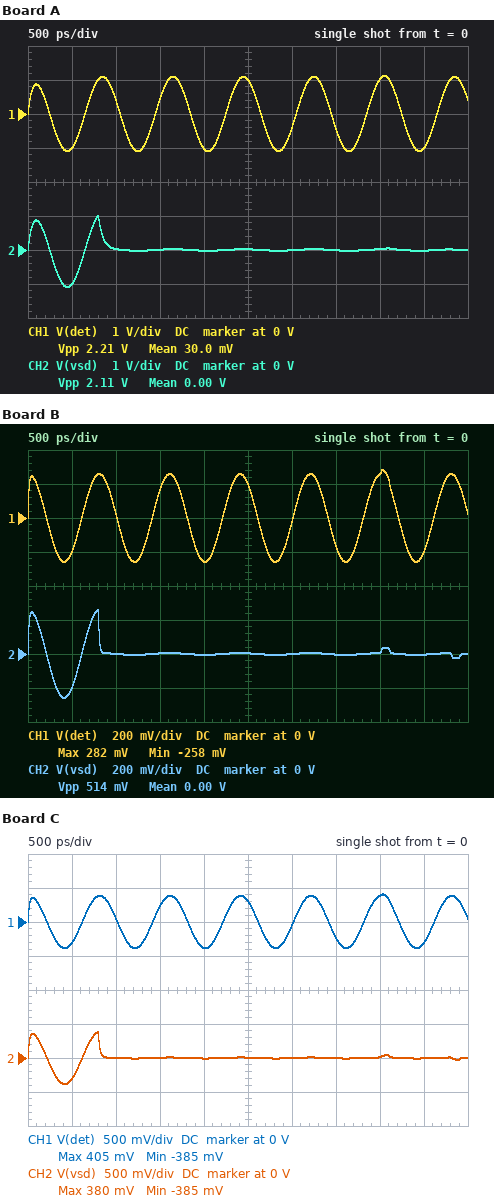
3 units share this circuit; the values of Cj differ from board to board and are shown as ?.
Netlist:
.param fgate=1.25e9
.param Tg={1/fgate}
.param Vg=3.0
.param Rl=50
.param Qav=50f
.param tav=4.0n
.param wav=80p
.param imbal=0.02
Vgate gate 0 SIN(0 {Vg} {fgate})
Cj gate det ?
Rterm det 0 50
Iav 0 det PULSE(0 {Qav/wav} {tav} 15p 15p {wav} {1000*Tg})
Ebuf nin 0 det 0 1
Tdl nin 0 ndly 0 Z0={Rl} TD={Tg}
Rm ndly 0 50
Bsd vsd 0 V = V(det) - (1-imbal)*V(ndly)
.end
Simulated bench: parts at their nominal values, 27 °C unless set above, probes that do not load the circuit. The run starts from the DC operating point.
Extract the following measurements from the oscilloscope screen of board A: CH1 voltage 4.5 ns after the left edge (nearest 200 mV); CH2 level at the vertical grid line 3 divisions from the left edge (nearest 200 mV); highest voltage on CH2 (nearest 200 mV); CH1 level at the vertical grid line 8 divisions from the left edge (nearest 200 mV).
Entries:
-1.0 V
0 V
1.0 V
1.0 V
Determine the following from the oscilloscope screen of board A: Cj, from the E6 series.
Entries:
1 pF
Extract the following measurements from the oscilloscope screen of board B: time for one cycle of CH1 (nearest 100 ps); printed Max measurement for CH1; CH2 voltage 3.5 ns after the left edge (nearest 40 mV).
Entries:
800 ps
282 mV
0 V
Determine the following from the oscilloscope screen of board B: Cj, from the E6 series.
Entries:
220 fF
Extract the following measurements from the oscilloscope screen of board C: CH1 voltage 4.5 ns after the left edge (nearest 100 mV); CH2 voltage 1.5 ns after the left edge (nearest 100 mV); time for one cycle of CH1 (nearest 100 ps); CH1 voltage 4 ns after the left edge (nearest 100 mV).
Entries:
-300 mV
0 V
800 ps
400 mV
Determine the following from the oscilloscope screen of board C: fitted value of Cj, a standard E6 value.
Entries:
330 fF
